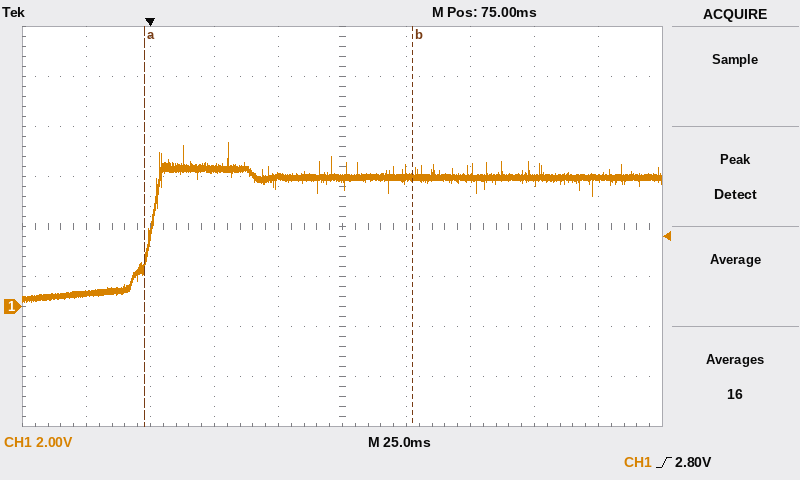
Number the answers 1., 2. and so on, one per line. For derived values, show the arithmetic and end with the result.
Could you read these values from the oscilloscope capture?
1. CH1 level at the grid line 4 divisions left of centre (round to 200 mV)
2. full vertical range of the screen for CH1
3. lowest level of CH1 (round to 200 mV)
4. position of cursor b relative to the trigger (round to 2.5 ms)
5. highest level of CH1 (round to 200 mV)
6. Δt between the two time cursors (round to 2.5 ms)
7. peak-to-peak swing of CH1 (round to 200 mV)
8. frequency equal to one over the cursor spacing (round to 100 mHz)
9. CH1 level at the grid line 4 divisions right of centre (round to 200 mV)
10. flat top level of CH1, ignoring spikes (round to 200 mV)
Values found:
1. 600 mV
2. 16 V
3. 200 mV
4. +102.5 ms
5. 6.6 V
6. 105.0 ms
7. 6.6 V − (200 mV) = 6.4 V
8. 1 / 105.0 ms ≈ 9.5 Hz
9. 5.2 V
10. 5.2 V
